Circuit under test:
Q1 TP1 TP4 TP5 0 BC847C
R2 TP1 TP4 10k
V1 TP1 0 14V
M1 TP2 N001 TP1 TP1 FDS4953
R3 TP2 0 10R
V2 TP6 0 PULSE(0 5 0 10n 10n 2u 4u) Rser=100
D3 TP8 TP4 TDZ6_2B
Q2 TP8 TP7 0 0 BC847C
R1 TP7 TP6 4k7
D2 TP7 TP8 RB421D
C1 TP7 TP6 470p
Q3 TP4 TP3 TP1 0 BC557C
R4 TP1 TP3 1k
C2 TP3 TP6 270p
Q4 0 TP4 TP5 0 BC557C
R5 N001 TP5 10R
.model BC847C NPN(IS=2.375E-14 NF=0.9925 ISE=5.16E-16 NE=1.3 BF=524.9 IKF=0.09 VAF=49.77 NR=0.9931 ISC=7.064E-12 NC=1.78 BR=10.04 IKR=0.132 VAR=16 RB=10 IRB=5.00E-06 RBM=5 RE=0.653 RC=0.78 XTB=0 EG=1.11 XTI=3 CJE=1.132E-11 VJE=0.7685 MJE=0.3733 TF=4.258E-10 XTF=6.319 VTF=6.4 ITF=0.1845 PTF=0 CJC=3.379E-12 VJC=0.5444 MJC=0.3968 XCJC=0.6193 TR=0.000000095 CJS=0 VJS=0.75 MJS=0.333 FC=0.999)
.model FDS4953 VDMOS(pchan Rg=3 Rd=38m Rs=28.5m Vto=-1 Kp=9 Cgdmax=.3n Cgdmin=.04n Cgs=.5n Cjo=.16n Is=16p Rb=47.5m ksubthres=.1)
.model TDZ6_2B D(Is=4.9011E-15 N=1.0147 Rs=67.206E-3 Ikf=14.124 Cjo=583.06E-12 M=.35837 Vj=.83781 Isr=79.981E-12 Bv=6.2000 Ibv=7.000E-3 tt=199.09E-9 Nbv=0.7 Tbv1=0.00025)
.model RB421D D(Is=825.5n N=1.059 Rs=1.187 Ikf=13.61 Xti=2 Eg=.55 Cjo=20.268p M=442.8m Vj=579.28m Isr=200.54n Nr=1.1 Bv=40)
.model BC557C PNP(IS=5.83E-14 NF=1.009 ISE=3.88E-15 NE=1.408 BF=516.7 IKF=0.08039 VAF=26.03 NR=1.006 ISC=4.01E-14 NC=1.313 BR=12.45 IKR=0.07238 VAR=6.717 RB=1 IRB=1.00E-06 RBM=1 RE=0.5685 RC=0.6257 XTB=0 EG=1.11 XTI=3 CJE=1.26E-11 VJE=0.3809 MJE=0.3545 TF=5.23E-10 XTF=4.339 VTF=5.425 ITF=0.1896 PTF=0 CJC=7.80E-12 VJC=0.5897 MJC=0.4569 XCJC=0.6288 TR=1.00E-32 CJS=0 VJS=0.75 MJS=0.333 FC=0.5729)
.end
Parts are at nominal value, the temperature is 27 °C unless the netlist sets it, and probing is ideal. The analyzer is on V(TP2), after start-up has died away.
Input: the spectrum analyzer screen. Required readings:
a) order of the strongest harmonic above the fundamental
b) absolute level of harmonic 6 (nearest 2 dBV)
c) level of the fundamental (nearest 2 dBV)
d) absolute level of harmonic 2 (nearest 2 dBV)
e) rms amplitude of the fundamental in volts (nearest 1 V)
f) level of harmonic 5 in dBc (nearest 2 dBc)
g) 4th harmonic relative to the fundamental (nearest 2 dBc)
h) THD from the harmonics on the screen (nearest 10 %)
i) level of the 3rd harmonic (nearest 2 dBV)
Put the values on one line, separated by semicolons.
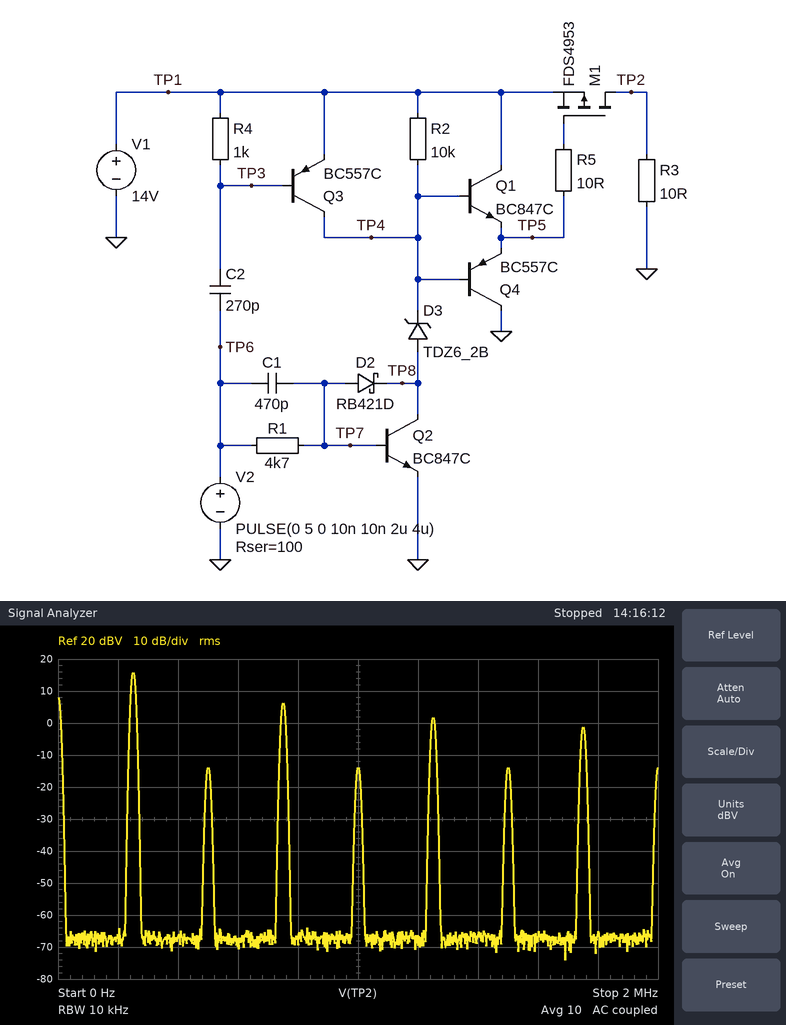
3; -14 dBV; 16 dBV; -14 dBV; 6 V; -14 dBc; -30 dBc; 40 %; 6 dBV
